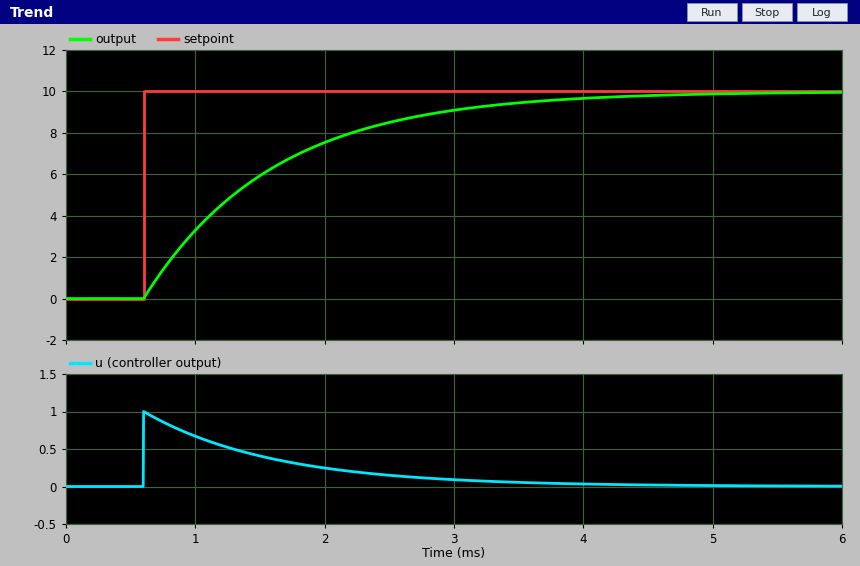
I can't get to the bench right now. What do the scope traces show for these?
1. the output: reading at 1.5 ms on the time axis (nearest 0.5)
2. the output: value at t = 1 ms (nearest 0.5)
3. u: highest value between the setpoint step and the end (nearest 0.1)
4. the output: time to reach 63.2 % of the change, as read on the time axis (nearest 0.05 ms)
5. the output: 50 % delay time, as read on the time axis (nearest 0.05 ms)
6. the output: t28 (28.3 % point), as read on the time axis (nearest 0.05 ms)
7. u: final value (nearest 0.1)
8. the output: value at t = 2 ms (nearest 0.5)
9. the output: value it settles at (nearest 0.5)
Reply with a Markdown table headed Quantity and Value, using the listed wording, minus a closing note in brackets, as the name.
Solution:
| Quantity | Value |
|---|---|
| the output: reading at 1.5 ms on the time axis | 6.0 |
| the output: value at t = 1 ms | 3.5 |
| u: highest value between the setpoint step and the end | 1.0 |
| the output: time to reach 63.2 % of the change, as read on the time axis | 1.60 ms |
| the output: 50 % delay time, as read on the time axis | 1.30 ms |
| the output: t28 (28.3 % point), as read on the time axis | 0.95 ms |
| u: final value | 0.0 |
| the output: value at t = 2 ms | 7.5 |
| the output: value it settles at | 10.0 |
